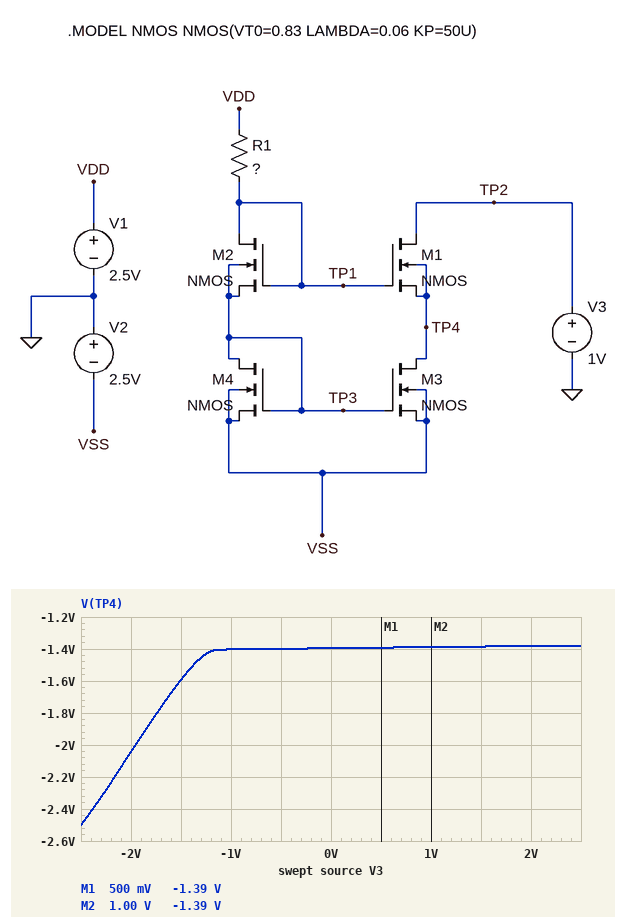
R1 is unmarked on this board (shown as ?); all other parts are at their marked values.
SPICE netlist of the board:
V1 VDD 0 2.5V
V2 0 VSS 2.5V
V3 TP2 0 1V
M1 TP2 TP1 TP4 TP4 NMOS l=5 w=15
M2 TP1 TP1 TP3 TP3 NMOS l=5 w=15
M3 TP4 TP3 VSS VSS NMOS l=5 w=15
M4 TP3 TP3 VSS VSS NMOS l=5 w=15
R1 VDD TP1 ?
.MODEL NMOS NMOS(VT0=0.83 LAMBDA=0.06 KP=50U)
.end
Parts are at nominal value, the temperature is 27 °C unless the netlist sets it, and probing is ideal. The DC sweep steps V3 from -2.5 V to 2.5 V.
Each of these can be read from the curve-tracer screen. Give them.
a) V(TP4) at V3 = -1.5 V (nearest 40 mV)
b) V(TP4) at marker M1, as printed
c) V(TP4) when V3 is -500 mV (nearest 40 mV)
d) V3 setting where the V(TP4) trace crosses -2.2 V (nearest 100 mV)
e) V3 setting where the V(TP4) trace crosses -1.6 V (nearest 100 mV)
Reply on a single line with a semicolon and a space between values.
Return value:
-1.60 V; -1.39 V; -1.40 V; -2.2 V; -1.5 V
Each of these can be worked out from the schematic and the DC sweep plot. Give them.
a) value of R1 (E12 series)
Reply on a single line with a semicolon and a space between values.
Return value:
470 kΩ
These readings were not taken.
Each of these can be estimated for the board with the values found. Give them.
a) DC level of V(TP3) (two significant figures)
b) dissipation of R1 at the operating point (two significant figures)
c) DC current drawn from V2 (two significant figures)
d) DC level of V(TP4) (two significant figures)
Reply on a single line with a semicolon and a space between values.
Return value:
-1.4 V; 17 µW; 12 µA; -1.4 V
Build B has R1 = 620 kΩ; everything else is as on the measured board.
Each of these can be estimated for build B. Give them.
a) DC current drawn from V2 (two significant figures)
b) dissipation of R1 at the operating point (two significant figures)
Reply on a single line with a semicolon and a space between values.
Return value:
9.2 µA; 13 µW
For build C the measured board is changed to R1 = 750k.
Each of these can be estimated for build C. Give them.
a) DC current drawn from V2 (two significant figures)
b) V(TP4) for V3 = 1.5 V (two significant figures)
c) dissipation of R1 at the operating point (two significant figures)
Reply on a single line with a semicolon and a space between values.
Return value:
7.7 µA; -1.4 V; 11 µW
